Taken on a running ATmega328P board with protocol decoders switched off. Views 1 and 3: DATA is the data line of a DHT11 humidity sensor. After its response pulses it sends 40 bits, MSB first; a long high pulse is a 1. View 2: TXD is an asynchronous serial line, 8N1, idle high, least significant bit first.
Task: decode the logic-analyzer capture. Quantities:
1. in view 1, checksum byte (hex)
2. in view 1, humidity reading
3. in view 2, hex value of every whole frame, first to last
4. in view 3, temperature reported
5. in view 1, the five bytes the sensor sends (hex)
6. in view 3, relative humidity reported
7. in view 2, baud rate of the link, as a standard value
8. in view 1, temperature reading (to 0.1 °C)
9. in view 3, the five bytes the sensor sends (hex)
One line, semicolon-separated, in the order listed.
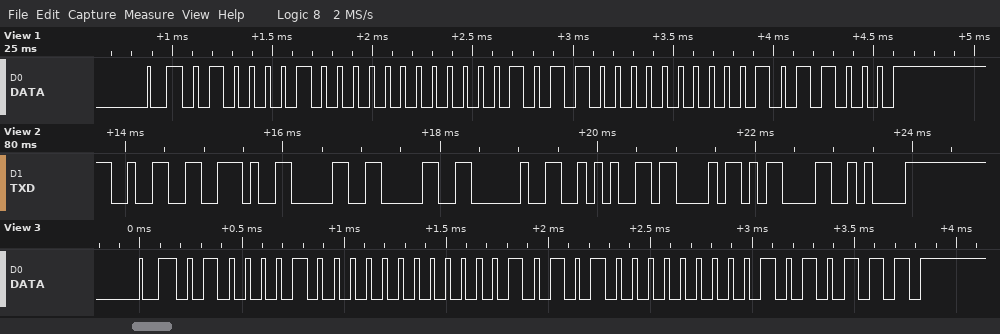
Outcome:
0x58; 66 %; 32 2E 30 30 20 2A 43 0D 0A; 21.0 °C; 42 00 16 00 58; 66 %; 9600 baud; 22.0 °C; 42 00 15 00 57
